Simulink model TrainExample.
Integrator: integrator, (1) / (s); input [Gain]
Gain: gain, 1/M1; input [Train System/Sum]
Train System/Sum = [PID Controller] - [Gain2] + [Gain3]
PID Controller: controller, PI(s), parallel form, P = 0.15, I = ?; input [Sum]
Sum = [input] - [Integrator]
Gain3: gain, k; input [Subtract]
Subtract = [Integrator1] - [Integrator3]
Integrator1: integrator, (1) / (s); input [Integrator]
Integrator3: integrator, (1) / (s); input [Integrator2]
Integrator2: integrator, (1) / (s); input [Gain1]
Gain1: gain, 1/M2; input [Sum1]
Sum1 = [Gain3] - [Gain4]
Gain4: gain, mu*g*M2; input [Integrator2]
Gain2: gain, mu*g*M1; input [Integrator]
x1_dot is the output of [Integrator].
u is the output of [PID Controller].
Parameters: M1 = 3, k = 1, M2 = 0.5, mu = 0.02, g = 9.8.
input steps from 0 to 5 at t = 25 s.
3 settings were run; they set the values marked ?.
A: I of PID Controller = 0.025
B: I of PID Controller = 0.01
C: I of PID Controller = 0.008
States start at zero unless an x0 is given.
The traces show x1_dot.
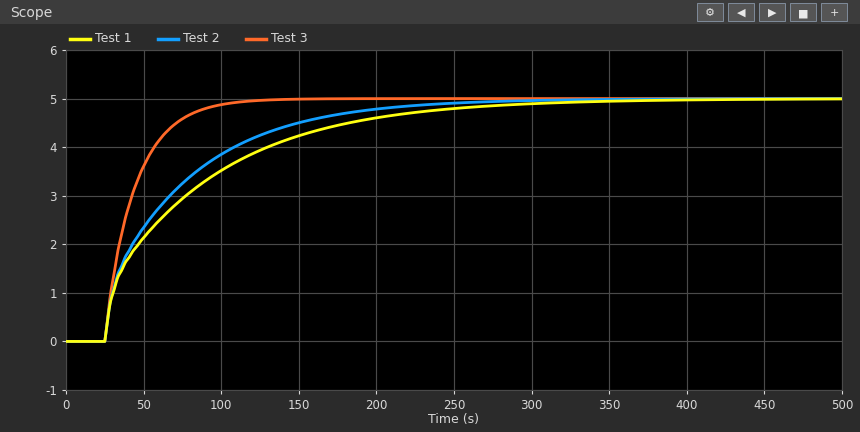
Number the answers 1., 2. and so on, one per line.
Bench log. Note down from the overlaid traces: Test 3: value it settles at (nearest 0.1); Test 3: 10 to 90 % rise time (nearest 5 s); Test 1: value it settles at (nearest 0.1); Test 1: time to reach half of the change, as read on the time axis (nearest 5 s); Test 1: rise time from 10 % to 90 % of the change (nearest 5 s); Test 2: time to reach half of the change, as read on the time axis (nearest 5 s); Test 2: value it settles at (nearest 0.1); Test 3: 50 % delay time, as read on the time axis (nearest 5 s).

1. 5.0
2. 45 s
3. 5.0
4. 60 s
5. 155 s
6. 55 s
7. 5.0
8. 40 s
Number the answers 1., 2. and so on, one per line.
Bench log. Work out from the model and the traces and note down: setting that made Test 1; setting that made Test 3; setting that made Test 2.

1. C
2. A
3. B
